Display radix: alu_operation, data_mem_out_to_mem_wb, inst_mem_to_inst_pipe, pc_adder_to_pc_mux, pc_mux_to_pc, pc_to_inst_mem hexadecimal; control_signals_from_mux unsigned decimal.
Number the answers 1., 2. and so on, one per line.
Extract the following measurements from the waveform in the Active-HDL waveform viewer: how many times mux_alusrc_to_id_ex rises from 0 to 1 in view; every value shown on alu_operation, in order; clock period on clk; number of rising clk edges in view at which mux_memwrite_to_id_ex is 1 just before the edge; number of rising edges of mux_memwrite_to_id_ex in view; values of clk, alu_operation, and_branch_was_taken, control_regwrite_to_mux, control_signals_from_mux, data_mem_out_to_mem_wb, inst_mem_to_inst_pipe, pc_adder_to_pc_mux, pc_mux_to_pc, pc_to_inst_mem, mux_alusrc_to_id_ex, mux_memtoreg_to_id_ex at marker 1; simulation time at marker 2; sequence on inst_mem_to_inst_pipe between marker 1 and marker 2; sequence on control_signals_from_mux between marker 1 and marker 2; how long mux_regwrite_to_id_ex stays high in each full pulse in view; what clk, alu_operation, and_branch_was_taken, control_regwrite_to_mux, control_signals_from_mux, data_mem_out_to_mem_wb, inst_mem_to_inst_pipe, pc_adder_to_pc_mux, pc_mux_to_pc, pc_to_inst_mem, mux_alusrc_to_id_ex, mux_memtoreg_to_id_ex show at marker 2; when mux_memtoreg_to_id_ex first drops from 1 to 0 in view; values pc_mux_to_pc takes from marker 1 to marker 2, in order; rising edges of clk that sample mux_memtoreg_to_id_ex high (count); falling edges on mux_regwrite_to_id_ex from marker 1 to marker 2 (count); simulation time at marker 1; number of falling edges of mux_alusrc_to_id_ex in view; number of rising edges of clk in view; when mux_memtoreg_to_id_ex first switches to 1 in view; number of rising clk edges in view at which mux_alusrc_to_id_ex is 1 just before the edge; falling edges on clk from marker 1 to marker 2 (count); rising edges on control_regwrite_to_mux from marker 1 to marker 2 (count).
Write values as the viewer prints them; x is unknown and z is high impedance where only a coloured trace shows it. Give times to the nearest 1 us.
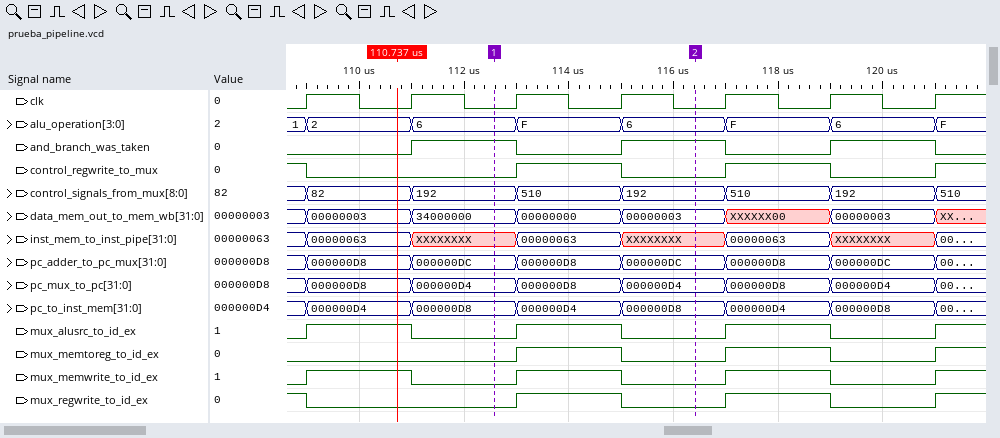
1. 4
2. 1, 2, 6, F, 6, F, 6, F
3. 2 us
4. 3
5. 4
6. clk=0, alu_operation=6, and_branch_was_taken=1, control_regwrite_to_mux=0, control_signals_from_mux=192, data_mem_out_to_mem_wb=34000000, inst_mem_to_inst_pipe=XXXXXXXX, pc_adder_to_pc_mux=000000DC, pc_mux_to_pc=000000D4, pc_to_inst_mem=000000D8, mux_alusrc_to_id_ex=0, mux_memtoreg_to_id_ex=0
7. 116 us
8. XXXXXXXX, 00000063, XXXXXXXX
9. 192, 510, 192
10. 2 us, 2 us
11. clk=0, alu_operation=6, and_branch_was_taken=1, control_regwrite_to_mux=0, control_signals_from_mux=192, data_mem_out_to_mem_wb=00000003, inst_mem_to_inst_pipe=XXXXXXXX, pc_adder_to_pc_mux=000000DC, pc_mux_to_pc=000000D4, pc_to_inst_mem=000000D8, mux_alusrc_to_id_ex=0, mux_memtoreg_to_id_ex=0
12. 115 us
13. 000000D4, 000000D8, 000000D4
14. 2
15. 1
16. 113 us
17. 3
18. 7
19. 113 us
20. 3
21. 2
22. 1
